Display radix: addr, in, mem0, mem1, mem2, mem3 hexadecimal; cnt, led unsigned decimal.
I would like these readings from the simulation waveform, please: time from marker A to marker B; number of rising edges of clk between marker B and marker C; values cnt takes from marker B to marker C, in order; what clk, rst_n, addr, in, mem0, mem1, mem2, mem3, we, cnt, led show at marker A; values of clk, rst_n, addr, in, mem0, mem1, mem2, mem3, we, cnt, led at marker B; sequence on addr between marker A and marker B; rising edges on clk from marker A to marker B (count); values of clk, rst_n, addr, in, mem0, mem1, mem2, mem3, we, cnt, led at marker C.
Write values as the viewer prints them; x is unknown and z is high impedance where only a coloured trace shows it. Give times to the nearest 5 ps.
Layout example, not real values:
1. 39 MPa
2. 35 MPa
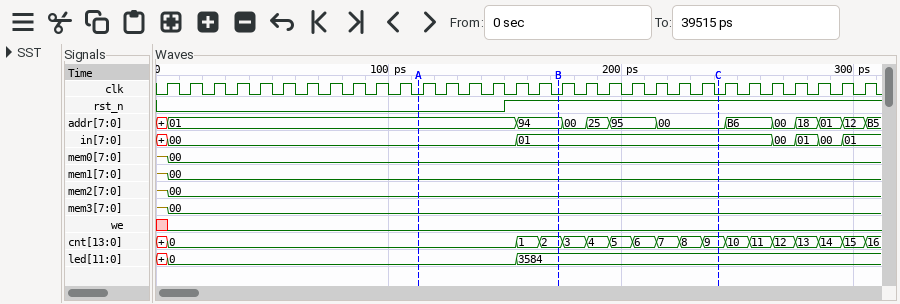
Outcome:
1. 60 ps
2. 7
3. 2, 3, 4, 5, 6, 7, 8, 9
4. clk=0, rst_n=0, addr=01, in=00, mem0=00, mem1=00, mem2=00, mem3=00, we=0, cnt=0, led=0
5. clk=0, rst_n=1, addr=94, in=01, mem0=00, mem1=00, mem2=00, mem3=00, we=0, cnt=2, led=3584
6. 01, 94
7. 6
8. clk=0, rst_n=1, addr=00, in=01, mem0=00, mem1=00, mem2=00, mem3=00, we=0, cnt=9, led=3584
